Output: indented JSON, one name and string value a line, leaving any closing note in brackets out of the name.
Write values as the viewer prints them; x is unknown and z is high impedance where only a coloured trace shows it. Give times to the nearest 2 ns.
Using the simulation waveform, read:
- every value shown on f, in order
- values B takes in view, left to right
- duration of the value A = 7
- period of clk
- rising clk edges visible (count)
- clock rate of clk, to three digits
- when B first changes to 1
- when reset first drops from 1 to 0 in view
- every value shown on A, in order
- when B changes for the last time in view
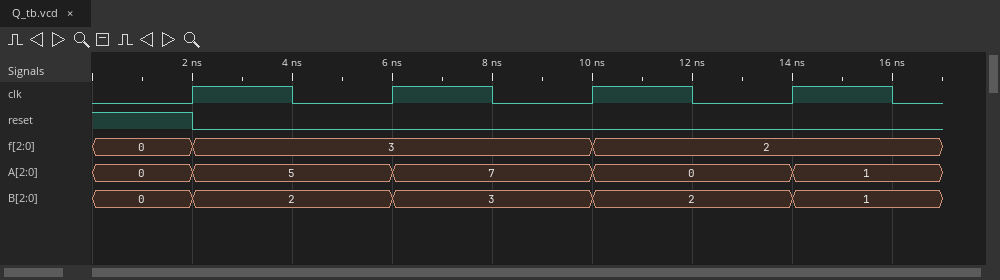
{
  "every value shown on f, in order": "0, 3, 2",
  "values B takes in view, left to right": "0, 2, 3, 2, 1",
  "duration of the value A = 7": "4 ns",
  "period of clk": "4 ns",
  "rising clk edges visible": "4",
  "clock rate of clk, to three digits": "250 MHz",
  "when B first changes to 1": "14 ns",
  "when reset first drops from 1 to 0 in view": "2 ns",
  "every value shown on A, in order": "0, 5, 7, 0, 1",
  "when B changes for the last time in view": "14 ns"
}
